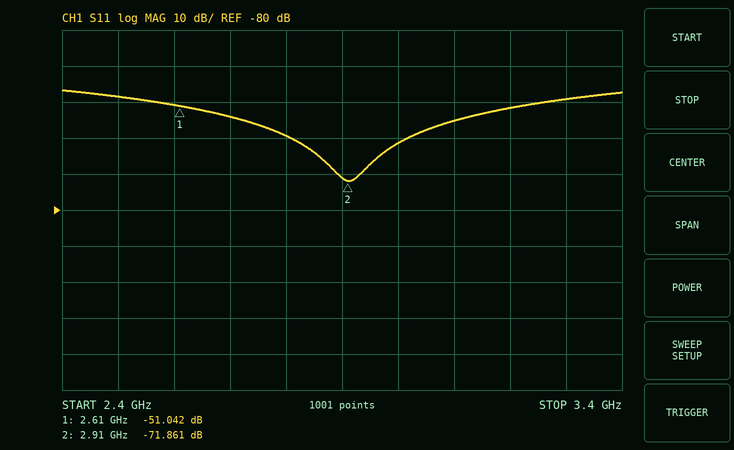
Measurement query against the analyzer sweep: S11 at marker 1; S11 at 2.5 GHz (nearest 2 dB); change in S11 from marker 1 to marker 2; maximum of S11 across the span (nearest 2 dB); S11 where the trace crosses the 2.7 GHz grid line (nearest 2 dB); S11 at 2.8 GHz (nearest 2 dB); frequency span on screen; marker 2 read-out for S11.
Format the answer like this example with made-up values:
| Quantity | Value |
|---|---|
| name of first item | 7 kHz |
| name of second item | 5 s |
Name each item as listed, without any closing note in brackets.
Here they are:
| Quantity | Value |
|---|---|
| S11 at marker 1 | -51.042 dB |
| S11 at 2.5 GHz | -48 dB |
| change in S11 from marker 1 to marker 2 | -20.819 dB |
| maximum of S11 across the span | -46 dB |
| S11 where the trace crosses the 2.7 GHz grid line | -54 dB |
| S11 at 2.8 GHz | -60 dB |
| frequency span on screen | 1 GHz |
| marker 2 read-out for S11 | -71.861 dB |
